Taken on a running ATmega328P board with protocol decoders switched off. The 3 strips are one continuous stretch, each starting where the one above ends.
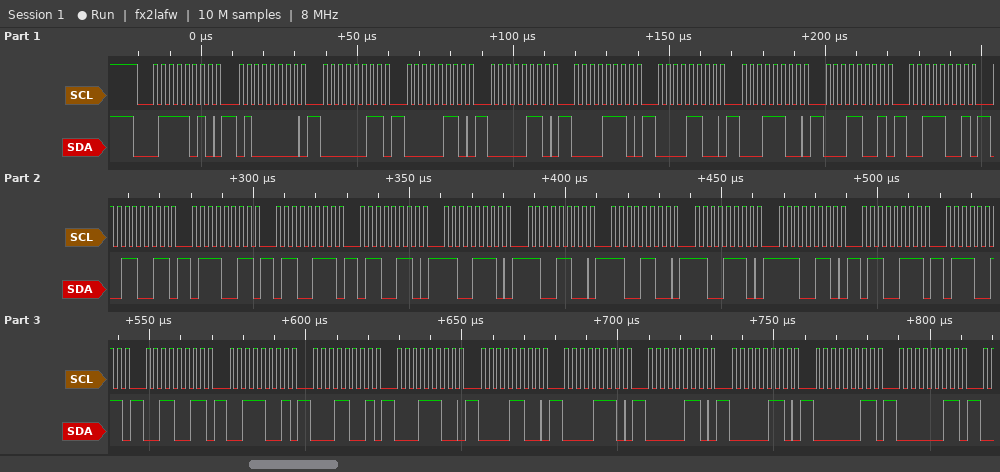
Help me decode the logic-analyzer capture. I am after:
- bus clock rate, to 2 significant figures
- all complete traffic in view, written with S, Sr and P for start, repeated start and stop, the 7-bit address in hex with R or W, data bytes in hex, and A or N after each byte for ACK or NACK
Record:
400 kHz
S 3DW A 40 A 03 A 06 A 06 A 0E A 0C A 1C A 19 A 39 A 33 A 73 A 67 A 66 A CE A CC A CC A CE A E6 A 67 A 73 A 33 A 39 A 19 A 1C A 0C A 0E A 06 A 06 A 03 A 03 A
